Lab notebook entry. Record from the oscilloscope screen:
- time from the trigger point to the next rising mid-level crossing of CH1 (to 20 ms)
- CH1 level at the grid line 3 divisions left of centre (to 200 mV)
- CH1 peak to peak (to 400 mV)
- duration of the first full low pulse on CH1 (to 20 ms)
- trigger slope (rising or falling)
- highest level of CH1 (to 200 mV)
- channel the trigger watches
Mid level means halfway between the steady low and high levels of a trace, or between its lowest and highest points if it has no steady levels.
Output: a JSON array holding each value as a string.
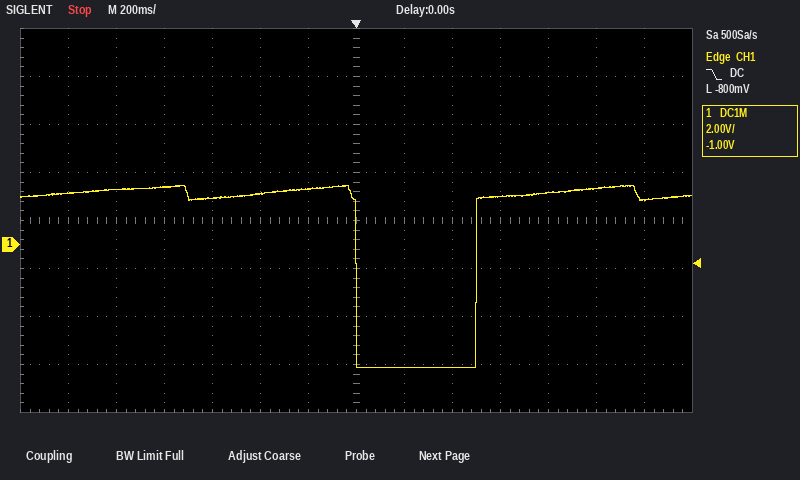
["500 ms", "2.0 V", "7.6 V", "500 ms", "falling", "2.4 V", "CH1"]
